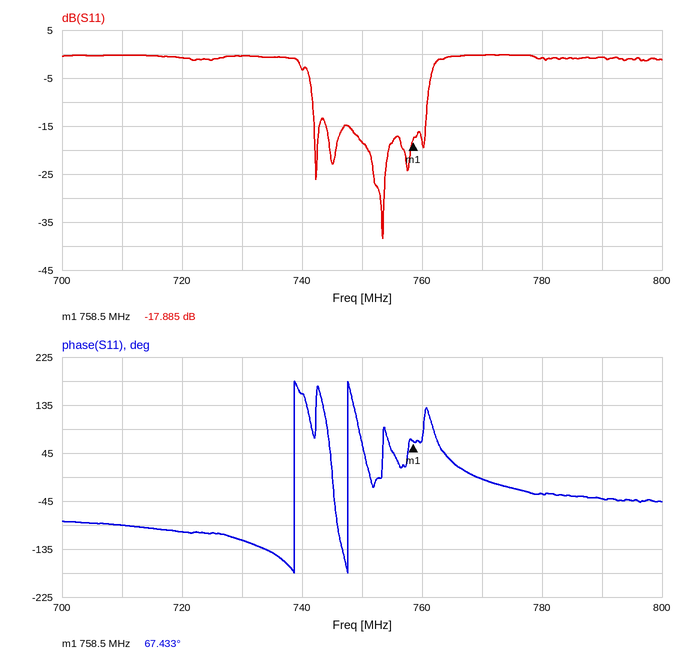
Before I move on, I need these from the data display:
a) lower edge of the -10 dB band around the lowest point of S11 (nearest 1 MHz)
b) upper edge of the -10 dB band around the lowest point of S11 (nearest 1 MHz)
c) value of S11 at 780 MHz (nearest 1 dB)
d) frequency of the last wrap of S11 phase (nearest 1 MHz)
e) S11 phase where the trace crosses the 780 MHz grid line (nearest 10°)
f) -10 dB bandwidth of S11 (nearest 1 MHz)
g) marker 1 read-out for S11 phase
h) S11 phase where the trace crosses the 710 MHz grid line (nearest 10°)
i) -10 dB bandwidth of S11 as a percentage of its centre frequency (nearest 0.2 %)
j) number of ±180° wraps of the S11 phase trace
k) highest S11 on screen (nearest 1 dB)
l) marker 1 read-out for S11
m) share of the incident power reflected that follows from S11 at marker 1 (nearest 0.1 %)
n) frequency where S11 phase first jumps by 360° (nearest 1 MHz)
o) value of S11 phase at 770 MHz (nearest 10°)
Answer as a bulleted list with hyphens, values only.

- 742 MHz
- 761 MHz
- -1 dB
- 748 MHz
- -30°
- 19 MHz
- 67.433°
- -90°
- 2.6 %
- 2
- 0 dB
- -17.885 dB
- 1.6 %
- 739 MHz
- 0°
